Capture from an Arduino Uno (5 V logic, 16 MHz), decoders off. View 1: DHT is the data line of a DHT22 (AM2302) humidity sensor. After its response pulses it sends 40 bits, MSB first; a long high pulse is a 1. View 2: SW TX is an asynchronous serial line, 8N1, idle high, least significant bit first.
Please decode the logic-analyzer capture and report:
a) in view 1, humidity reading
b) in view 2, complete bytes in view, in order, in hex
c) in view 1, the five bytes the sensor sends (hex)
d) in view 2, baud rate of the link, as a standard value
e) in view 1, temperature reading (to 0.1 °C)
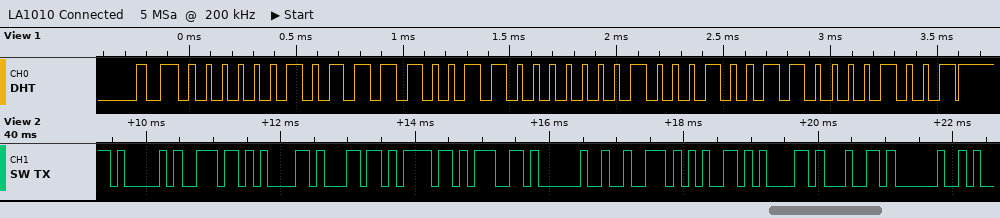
75.5 %
0x41 0x6E 0x61 0x6C 0x6F 0x67 0x20 0x72 0x65 0x61 0x64 0x20
02 F3 01 13 09
9600 baud
27.5 °C
